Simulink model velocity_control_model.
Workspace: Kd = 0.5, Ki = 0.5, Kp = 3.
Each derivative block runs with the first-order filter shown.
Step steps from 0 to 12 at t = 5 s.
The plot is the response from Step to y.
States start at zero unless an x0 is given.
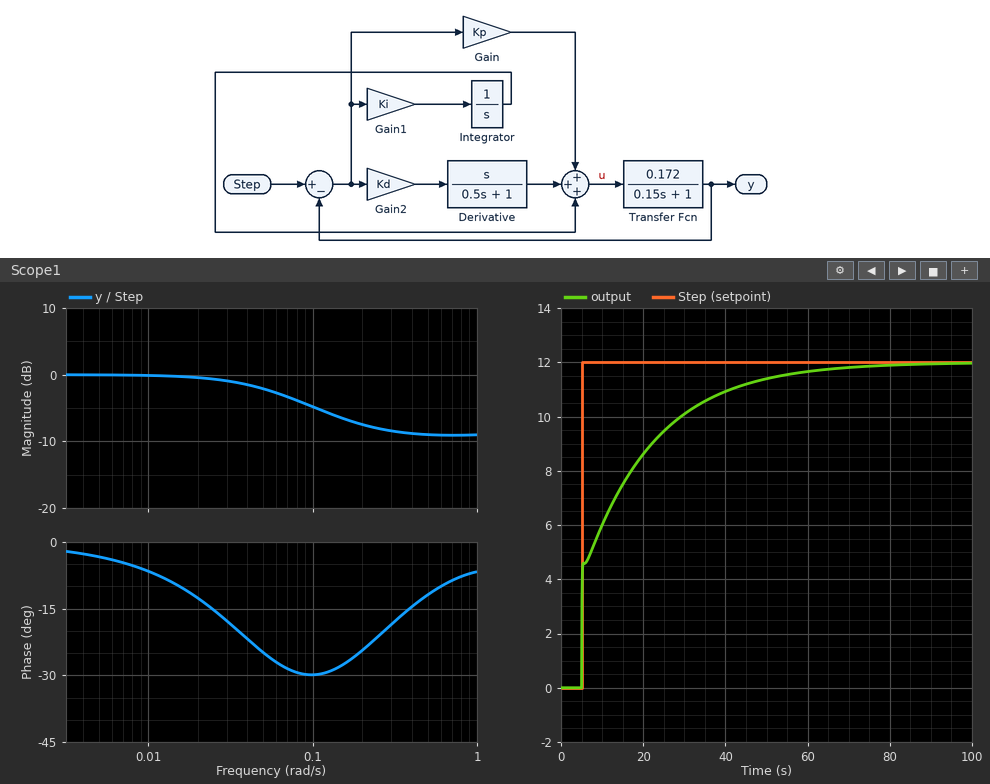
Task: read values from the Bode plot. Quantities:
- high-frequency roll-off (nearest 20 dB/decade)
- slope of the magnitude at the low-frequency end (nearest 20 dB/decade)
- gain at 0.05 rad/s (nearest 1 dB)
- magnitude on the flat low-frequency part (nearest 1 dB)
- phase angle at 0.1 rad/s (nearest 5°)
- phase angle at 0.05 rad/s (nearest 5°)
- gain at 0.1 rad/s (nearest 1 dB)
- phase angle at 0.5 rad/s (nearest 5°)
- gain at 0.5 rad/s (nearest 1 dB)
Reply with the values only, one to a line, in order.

0 dB/decade
0 dB/decade
-2 dB
0 dB
-30°
-25°
-5 dB
-10°
-9 dB
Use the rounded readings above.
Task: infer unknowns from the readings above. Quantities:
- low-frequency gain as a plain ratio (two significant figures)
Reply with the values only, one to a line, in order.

1.0
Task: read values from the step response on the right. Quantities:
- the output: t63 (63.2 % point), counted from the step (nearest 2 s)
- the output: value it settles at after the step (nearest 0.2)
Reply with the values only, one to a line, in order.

10 s
12.0
